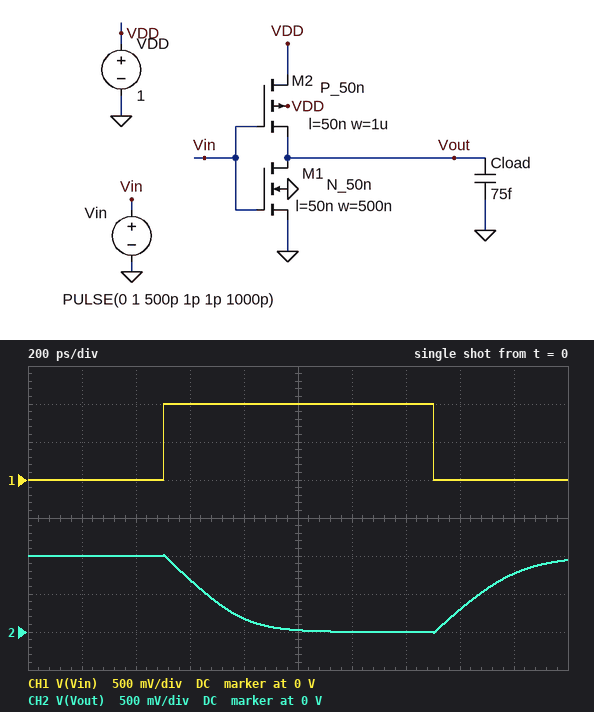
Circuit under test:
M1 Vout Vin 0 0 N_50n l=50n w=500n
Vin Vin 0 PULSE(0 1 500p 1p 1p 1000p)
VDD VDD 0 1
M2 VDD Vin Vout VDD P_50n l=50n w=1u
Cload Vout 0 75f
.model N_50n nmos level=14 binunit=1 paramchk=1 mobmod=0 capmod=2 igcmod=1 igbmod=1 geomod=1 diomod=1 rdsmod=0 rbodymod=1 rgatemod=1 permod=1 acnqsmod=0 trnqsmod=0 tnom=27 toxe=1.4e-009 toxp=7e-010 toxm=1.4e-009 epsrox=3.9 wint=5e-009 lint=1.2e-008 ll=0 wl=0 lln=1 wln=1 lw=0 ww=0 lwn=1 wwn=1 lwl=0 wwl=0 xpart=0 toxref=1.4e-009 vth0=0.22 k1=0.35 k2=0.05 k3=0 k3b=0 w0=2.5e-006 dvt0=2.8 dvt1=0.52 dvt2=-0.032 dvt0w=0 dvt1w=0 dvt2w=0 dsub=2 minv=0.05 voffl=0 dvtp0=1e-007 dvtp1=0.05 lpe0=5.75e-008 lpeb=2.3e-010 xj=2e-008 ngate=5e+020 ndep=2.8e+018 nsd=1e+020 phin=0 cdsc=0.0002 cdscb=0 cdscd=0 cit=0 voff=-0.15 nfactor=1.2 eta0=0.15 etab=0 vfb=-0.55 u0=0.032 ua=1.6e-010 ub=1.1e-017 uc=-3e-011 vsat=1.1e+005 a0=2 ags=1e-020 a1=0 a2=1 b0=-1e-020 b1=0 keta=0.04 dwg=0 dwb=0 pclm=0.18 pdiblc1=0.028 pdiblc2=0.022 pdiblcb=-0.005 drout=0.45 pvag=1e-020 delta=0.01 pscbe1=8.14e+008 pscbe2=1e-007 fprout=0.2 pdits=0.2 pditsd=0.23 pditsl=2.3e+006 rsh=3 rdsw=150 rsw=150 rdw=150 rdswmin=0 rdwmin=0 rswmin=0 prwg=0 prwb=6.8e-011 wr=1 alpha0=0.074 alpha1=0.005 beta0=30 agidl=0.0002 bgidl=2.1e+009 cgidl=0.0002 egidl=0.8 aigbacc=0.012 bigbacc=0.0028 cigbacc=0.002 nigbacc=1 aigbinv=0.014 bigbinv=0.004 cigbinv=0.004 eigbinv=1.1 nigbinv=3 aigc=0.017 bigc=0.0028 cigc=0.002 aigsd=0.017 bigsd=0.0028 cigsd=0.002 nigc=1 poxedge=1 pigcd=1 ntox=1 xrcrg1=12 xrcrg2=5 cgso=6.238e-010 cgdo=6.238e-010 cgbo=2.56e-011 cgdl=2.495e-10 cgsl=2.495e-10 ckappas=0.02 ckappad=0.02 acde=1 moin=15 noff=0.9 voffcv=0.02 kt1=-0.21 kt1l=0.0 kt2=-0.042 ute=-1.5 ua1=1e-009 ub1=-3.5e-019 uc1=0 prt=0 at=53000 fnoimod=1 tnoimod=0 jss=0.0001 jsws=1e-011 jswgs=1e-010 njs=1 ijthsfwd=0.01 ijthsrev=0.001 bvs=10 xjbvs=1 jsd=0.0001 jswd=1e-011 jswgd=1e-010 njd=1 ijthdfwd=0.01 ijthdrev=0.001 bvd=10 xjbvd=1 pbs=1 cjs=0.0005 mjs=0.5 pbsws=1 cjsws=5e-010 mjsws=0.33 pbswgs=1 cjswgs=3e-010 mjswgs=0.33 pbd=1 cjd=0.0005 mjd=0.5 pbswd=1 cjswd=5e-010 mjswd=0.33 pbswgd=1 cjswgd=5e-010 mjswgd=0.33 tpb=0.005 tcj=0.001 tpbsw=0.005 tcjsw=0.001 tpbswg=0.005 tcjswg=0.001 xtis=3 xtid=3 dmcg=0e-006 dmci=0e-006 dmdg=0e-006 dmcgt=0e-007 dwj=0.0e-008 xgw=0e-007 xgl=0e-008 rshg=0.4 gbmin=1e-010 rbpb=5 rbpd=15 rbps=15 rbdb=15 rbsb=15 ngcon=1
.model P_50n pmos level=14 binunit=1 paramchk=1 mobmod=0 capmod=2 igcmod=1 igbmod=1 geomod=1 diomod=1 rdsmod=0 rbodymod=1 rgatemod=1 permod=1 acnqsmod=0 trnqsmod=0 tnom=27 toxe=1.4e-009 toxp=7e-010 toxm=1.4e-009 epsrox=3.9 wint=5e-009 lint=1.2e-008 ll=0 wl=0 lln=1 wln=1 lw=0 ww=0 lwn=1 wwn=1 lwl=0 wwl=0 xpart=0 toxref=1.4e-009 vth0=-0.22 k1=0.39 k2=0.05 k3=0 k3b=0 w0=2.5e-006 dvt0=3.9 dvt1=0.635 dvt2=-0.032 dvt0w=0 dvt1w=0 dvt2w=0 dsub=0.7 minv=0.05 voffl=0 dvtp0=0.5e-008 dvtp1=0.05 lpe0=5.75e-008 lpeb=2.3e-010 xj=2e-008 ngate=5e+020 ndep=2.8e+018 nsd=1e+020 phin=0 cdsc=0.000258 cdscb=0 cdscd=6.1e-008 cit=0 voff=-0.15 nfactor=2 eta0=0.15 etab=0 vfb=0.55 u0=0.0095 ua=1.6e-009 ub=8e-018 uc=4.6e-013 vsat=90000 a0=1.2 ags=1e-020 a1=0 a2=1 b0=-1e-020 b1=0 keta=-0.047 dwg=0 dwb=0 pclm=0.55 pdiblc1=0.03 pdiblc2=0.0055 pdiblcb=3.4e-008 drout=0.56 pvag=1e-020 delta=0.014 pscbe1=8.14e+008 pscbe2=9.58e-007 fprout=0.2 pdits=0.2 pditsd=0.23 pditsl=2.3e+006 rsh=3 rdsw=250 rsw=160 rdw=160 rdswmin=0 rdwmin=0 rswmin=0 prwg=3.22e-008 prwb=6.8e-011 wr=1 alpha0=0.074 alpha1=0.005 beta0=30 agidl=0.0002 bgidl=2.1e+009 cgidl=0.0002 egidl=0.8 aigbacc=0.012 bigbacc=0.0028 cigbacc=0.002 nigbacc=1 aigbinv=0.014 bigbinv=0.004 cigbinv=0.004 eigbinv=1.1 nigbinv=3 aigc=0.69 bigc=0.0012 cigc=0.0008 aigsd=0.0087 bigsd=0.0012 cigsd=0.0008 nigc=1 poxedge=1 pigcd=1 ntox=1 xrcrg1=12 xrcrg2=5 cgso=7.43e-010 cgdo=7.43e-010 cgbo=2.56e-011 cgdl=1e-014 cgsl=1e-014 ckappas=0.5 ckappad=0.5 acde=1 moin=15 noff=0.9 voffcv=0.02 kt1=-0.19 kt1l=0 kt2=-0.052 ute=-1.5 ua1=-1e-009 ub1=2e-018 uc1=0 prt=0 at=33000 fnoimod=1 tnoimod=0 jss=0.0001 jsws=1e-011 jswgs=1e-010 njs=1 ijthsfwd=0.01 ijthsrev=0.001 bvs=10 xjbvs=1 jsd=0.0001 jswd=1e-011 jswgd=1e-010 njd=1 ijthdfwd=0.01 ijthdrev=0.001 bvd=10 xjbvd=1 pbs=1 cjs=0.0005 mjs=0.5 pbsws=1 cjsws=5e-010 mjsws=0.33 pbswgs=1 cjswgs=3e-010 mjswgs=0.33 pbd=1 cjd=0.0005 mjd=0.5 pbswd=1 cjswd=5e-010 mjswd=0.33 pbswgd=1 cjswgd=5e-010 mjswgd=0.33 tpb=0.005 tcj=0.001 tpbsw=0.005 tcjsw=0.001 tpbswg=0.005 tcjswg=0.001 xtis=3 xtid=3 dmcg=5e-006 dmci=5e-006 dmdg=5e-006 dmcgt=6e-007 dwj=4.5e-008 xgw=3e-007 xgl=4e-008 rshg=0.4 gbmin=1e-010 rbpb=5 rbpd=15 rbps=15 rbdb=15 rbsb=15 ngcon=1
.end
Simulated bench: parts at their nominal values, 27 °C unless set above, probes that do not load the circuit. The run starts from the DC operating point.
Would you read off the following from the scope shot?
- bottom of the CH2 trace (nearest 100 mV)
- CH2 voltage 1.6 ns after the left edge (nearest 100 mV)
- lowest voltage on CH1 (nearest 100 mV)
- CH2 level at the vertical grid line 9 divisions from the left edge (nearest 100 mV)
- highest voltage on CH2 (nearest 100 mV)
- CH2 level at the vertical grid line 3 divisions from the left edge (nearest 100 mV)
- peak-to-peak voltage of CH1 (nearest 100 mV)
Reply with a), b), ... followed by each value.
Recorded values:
a) 0 V
b) 300 mV
c) 0 V
d) 800 mV
e) 1.0 V
f) 700 mV
g) 1.0 V
